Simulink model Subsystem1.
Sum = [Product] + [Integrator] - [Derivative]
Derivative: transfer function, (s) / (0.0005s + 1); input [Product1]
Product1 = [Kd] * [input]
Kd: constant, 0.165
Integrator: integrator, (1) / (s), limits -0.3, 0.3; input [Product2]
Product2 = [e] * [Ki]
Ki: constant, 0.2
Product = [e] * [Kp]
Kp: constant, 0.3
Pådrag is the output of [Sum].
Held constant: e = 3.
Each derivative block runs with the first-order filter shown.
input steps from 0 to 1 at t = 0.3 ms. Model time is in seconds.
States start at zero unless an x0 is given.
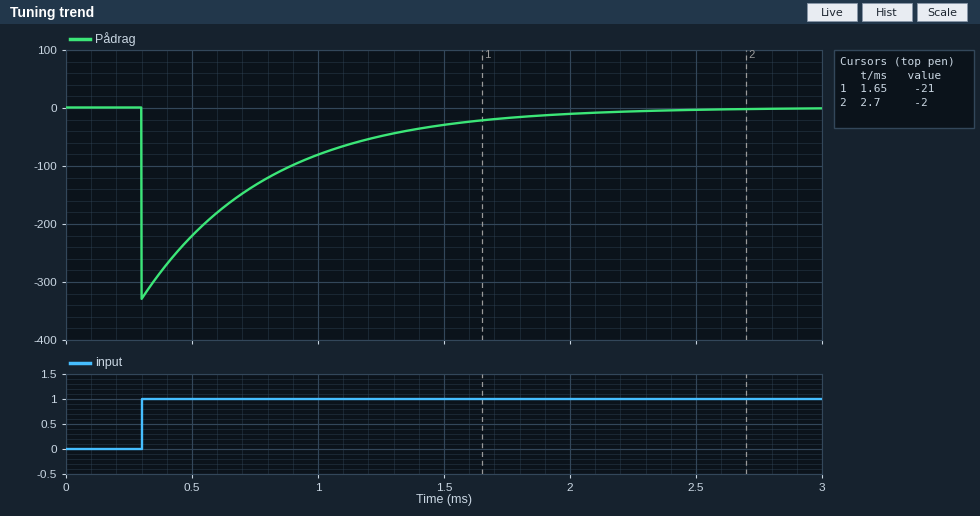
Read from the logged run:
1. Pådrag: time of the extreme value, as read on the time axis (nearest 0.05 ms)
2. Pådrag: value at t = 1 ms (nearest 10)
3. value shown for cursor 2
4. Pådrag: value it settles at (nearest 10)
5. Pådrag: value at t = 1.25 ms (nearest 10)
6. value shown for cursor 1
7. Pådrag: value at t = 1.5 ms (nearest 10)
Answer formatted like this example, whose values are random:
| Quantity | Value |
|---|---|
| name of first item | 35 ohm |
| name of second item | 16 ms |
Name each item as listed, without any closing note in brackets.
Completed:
| Quantity | Value |
|---|---|
| Pådrag: time of the extreme value, as read on the time axis | 0.30 ms |
| Pådrag: value at t = 1 ms | -80 |
| value shown for cursor 2 | -2 |
| Pådrag: value it settles at | 0 |
| Pådrag: value at t = 1.25 ms | -50 |
| value shown for cursor 1 | -21 |
| Pådrag: value at t = 1.5 ms | -30 |
